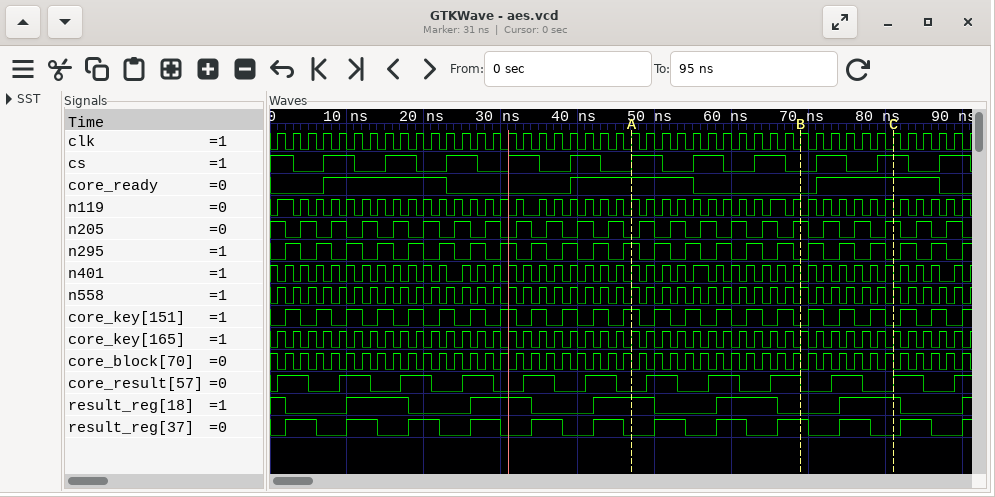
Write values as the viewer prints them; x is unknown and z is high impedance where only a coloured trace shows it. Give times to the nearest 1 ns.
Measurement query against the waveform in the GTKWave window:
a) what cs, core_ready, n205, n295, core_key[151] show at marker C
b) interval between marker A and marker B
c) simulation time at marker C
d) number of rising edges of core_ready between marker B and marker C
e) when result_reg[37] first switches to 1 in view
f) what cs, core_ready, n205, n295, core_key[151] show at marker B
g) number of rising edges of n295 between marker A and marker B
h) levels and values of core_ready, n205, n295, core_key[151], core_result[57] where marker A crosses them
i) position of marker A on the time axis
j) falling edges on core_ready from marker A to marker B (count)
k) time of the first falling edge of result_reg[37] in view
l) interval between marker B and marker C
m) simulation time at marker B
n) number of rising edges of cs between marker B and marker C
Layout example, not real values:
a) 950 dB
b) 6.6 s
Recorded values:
a) cs=1, core_ready=1, n205=1, n295=0, core_key[151]=0
b) 22 ns
c) 81 ns
d) 1
e) 2 ns
f) cs=0, core_ready=0, n205=1, n295=0, core_key[151]=0
g) 5
h) core_ready=1, n205=0, n295=1, core_key[151]=1, core_result[57]=0
i) 47 ns
j) 1
k) 6 ns
l) 12 ns
m) 69 ns
n) 2
